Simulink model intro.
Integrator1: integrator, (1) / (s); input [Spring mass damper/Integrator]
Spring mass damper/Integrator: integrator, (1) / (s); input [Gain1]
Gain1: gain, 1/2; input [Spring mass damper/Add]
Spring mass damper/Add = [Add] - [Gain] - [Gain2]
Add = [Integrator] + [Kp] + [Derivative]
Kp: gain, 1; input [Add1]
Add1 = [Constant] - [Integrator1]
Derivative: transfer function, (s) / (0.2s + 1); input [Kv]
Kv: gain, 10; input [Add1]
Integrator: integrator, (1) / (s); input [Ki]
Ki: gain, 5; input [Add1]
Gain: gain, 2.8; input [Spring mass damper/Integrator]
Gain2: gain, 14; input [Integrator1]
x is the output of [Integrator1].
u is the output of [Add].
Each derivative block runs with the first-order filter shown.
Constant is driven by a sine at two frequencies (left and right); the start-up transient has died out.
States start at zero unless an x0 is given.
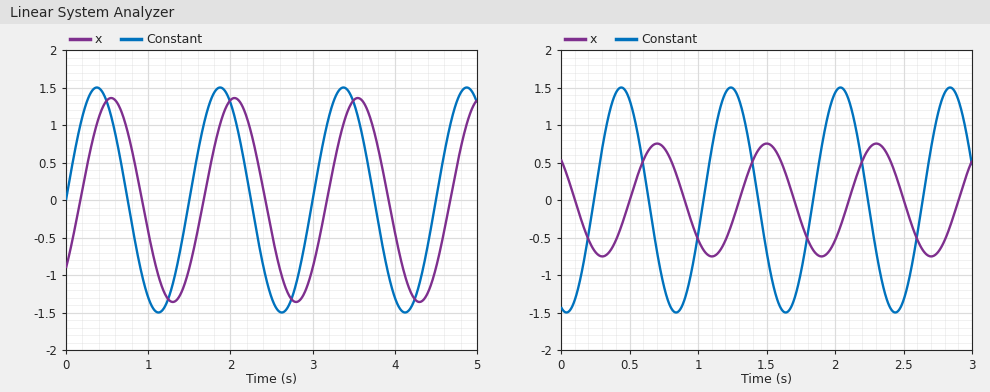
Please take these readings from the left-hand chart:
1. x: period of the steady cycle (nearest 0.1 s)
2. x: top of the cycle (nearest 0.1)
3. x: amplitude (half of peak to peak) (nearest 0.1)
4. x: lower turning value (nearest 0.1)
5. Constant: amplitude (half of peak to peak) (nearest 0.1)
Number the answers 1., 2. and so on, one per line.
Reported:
1. 1.5 s
2. 1.4
3. 1.4
4. -1.4
5. 1.5
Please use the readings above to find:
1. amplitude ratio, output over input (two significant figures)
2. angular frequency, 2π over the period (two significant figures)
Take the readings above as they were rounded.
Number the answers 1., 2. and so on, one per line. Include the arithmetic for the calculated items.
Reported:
1. 1.4 / 1.5 = 0.93
2. 2π / 1.5 = 4.2 rad/s
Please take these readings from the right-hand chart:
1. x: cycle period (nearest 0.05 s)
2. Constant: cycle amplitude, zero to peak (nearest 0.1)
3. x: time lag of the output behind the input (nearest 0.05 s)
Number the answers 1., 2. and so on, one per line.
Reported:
1. 0.80 s
2. 1.5
3. 0.25 s
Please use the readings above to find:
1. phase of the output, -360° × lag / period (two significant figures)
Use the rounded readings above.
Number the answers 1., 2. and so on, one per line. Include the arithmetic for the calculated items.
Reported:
1. -360 × 0.25 / 0.8 = -110°
